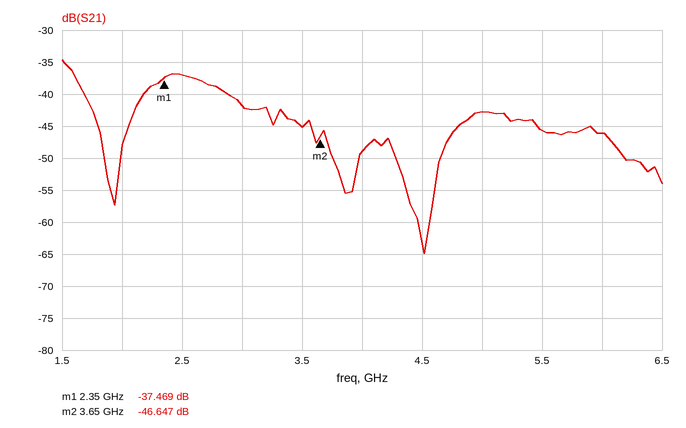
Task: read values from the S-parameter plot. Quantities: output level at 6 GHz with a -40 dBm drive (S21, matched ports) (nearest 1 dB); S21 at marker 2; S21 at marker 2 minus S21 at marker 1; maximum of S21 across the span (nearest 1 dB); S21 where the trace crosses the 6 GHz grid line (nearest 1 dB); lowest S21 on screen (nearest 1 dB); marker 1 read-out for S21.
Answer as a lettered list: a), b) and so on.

a) -86 dBm
b) -46.647 dB
c) -9.178 dB
d) -35 dB
e) -46 dB
f) -65 dB
g) -37.469 dB
